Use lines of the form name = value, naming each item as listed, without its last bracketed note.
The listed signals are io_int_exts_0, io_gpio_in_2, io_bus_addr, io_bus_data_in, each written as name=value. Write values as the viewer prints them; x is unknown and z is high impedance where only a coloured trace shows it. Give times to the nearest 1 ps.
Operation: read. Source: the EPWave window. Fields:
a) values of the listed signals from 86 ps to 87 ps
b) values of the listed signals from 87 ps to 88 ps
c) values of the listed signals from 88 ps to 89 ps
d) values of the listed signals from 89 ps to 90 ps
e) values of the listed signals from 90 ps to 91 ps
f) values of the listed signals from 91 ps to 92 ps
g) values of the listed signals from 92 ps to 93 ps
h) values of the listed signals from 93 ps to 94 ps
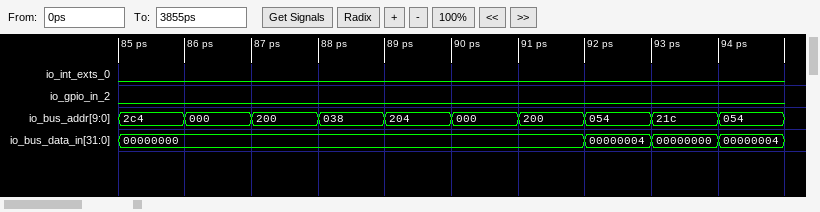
values of the listed signals from 86 ps to 87 ps = io_int_exts_0=0, io_gpio_in_2=0, io_bus_addr=000, io_bus_data_in=00000000
values of the listed signals from 87 ps to 88 ps = io_int_exts_0=0, io_gpio_in_2=0, io_bus_addr=200, io_bus_data_in=00000000
values of the listed signals from 88 ps to 89 ps = io_int_exts_0=0, io_gpio_in_2=0, io_bus_addr=038, io_bus_data_in=00000000
values of the listed signals from 89 ps to 90 ps = io_int_exts_0=0, io_gpio_in_2=0, io_bus_addr=204, io_bus_data_in=00000000
values of the listed signals from 90 ps to 91 ps = io_int_exts_0=0, io_gpio_in_2=0, io_bus_addr=000, io_bus_data_in=00000000
values of the listed signals from 91 ps to 92 ps = io_int_exts_0=0, io_gpio_in_2=0, io_bus_addr=200, io_bus_data_in=00000000
values of the listed signals from 92 ps to 93 ps = io_int_exts_0=0, io_gpio_in_2=0, io_bus_addr=054, io_bus_data_in=00000004
values of the listed signals from 93 ps to 94 ps = io_int_exts_0=0, io_gpio_in_2=0, io_bus_addr=21c, io_bus_data_in=00000000
